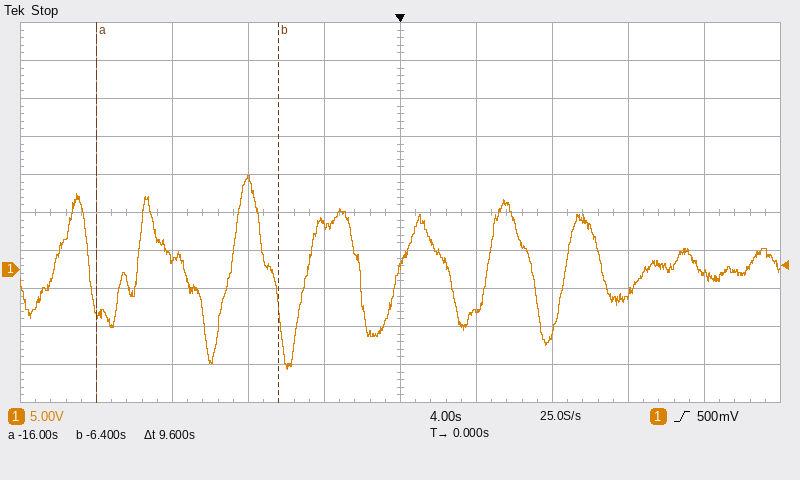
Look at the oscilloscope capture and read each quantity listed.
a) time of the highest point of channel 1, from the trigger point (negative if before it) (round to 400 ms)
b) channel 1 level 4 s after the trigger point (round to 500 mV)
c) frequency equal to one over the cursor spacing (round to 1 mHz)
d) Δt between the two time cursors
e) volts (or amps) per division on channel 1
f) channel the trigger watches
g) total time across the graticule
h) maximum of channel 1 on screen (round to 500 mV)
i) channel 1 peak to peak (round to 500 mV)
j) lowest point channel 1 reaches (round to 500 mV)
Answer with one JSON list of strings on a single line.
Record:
["-8.0 s", "-5.5 V", "104 mHz", "9.6 s", "5 V", "channel 1", "40 s", "12.5 V", "25.5 V", "-13.0 V"]
